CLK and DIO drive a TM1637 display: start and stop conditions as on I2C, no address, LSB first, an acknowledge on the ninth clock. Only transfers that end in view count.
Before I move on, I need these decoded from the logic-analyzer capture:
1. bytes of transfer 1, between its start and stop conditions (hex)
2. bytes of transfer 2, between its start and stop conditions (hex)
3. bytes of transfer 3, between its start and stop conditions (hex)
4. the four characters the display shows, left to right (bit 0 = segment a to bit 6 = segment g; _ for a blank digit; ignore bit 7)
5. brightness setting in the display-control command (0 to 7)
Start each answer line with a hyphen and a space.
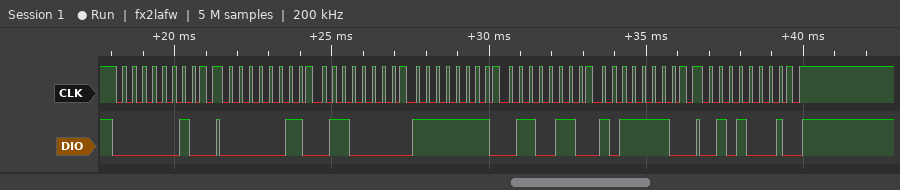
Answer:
- 40
- C0 06 FF 66 7D
- 8A
- 1846
- 2
